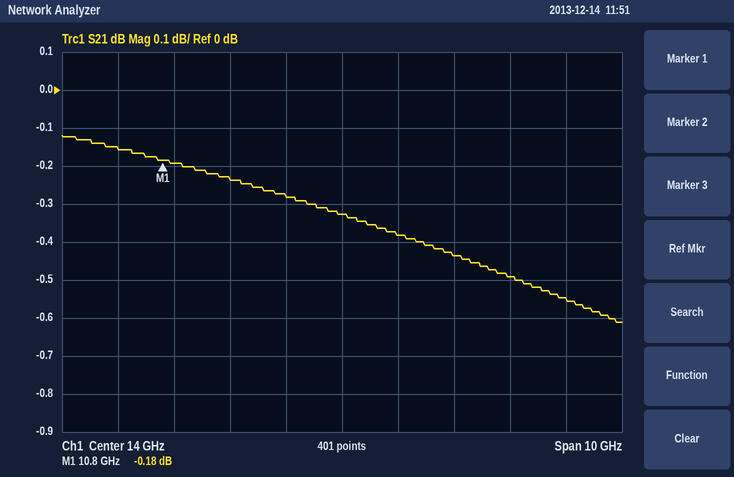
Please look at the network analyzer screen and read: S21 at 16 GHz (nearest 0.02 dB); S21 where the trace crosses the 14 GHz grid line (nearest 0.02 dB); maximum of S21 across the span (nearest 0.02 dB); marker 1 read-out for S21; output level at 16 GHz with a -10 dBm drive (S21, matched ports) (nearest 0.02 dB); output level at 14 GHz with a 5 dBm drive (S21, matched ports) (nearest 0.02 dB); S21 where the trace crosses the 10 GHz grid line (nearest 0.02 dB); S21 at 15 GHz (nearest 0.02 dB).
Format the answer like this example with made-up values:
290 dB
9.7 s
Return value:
-0.44 dB
-0.32 dB
-0.12 dB
-0.18 dB
-10.44 dBm
4.68 dBm
-0.16 dB
-0.38 dB
